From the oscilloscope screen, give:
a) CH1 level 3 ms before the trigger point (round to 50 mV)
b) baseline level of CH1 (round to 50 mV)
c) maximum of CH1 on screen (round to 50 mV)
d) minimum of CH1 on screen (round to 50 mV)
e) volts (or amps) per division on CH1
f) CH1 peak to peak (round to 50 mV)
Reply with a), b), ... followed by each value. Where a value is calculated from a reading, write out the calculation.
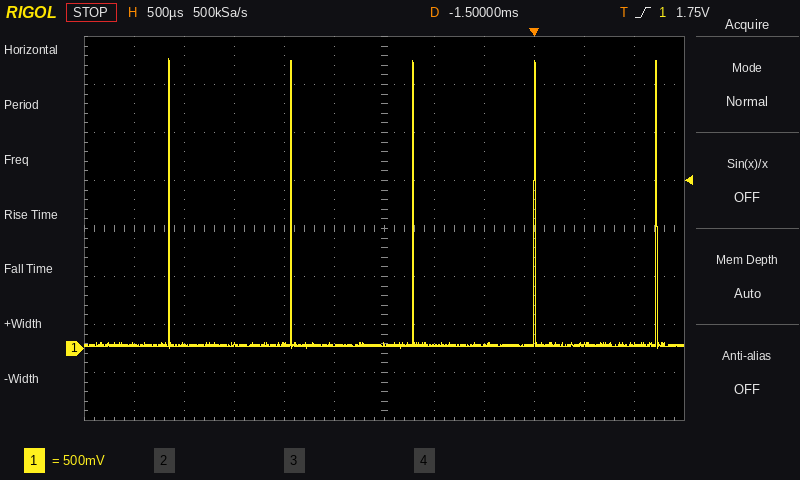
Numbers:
a) 50 mV
b) 50 mV
c) 3.00 V
d) 0 mV
e) 500 mV
f) 3.00 V − (0 mV) = 3.00 V
